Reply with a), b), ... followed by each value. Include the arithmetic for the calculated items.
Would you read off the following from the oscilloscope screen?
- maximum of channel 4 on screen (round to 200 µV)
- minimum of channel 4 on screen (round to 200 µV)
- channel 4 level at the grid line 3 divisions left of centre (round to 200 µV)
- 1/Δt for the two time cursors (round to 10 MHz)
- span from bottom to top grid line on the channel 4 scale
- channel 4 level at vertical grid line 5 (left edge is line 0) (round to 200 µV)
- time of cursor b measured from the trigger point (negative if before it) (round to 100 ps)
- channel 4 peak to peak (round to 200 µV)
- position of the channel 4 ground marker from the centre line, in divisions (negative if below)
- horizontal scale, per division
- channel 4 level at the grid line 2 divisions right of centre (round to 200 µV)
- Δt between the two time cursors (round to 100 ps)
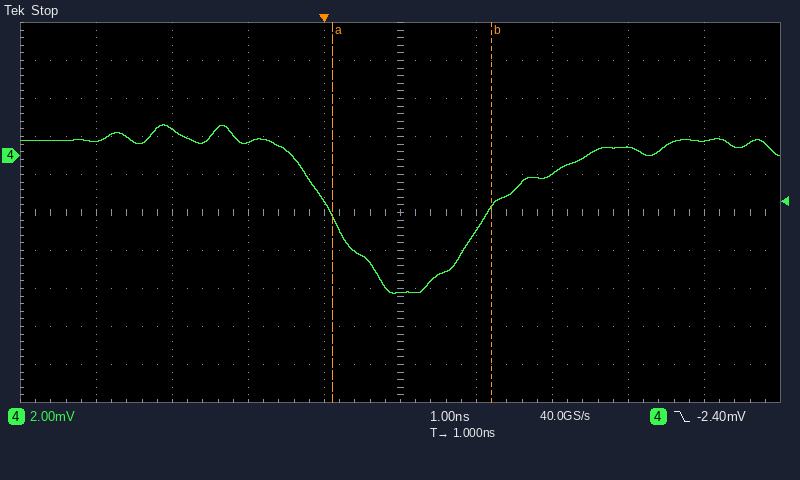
a) 1.6 mV
b) -7.2 mV
c) 1.4 mV
d) 1 / 2.1 ns ≈ 480 MHz
e) 20 mV
f) -7.2 mV
g) +2.2 ns
h) 1.6 mV − (-7.2 mV) = 8.8 mV
i) +1.5 div
j) 1 ns
k) -1.0 mV
l) 2.1 ns
